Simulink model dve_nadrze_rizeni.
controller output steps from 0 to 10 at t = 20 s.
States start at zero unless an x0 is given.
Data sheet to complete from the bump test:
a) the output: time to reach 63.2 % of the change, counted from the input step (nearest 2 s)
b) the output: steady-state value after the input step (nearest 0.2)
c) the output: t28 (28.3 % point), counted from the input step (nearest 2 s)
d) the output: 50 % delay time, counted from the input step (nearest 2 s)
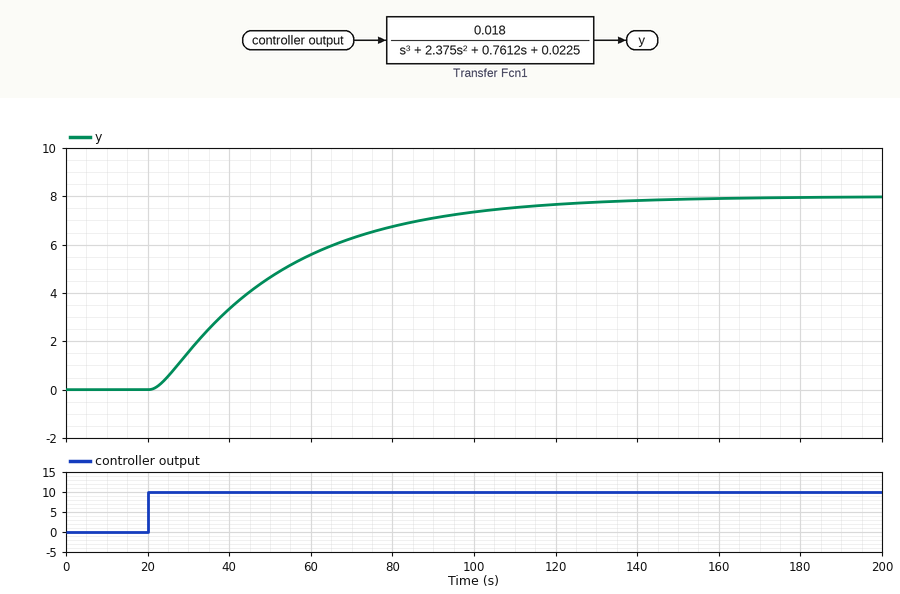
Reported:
34 s
8.0
14 s
24 s
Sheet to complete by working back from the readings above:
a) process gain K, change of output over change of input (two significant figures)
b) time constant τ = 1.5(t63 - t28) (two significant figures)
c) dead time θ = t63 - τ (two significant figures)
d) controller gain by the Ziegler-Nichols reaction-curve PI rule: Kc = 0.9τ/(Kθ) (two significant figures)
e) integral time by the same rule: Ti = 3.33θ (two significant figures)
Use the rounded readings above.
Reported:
0.80
30 s
4.0 s
8.4
13 s
